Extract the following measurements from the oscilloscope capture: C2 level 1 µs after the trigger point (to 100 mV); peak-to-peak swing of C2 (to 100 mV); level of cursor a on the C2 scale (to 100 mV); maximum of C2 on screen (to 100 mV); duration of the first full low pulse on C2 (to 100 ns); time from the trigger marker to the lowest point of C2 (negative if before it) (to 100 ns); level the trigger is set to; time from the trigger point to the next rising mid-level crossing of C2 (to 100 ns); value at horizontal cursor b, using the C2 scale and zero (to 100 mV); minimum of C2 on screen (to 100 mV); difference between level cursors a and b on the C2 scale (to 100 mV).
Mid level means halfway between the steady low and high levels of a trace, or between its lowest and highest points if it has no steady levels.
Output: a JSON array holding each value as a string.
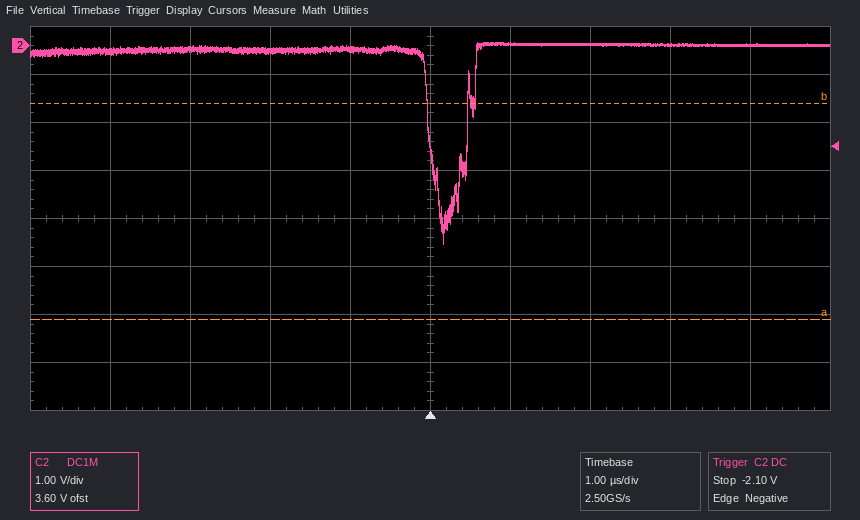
["0.0 V", "4.2 V", "-5.7 V", "100 mV", "500 ns", "+200 ns", "-2.10 V", "500 ns", "-1.2 V", "-4.1 V", "4.5 V"]
